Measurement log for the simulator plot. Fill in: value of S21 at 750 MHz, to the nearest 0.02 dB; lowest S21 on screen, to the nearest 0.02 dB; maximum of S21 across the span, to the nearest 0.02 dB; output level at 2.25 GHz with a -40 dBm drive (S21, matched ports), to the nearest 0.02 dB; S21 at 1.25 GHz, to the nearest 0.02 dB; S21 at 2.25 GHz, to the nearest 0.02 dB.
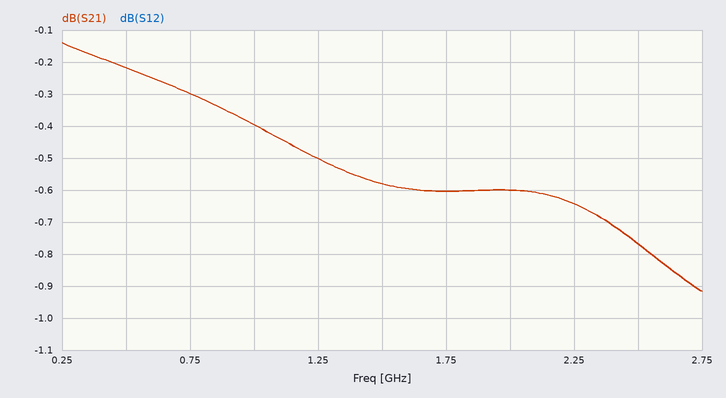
-0.30 dB
-0.92 dB
-0.14 dB
-40.64 dBm
-0.50 dB
-0.64 dB
